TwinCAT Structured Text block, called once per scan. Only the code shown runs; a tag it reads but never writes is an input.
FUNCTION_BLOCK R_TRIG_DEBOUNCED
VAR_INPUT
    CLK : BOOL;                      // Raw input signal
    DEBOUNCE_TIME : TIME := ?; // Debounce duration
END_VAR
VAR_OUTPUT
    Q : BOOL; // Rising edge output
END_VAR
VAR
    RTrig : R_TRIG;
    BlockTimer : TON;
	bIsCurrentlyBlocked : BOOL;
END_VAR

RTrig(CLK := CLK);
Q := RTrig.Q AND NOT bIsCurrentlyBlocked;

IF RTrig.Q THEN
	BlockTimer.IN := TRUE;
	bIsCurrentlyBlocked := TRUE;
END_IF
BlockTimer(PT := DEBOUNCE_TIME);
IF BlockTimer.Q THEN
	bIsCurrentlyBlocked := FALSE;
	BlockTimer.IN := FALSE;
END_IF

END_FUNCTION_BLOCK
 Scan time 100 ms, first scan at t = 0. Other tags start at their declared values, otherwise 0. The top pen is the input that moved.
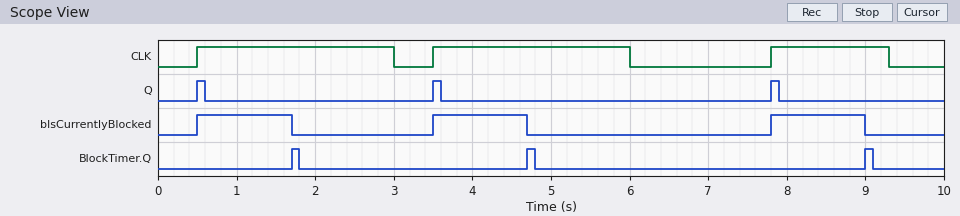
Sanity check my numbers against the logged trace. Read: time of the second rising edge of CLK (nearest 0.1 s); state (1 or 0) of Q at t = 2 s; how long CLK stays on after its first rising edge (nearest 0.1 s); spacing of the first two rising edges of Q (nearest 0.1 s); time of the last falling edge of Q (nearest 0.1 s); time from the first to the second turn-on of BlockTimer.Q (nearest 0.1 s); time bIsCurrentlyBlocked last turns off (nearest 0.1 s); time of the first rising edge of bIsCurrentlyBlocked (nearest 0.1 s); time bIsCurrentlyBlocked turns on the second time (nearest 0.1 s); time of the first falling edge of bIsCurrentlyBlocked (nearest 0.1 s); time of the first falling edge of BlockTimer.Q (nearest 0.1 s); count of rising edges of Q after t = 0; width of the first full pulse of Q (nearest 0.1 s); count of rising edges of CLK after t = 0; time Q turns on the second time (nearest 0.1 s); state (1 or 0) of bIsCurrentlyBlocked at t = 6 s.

3.5 s
0
2.5 s
3.0 s
7.9 s
3.0 s
9.0 s
0.5 s
3.5 s
1.7 s
1.8 s
3
0.1 s
3
3.5 s
0
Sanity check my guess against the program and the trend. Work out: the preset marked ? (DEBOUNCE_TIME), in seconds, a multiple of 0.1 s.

1.2 s
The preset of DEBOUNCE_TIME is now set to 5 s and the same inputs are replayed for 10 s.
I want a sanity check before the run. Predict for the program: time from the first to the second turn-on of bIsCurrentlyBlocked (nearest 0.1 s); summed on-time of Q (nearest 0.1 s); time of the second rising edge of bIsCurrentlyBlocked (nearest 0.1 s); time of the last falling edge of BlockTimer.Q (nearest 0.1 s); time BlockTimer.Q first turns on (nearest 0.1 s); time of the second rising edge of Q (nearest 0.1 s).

7.3 s
0.2 s
7.8 s
5.6 s
5.5 s
7.8 s
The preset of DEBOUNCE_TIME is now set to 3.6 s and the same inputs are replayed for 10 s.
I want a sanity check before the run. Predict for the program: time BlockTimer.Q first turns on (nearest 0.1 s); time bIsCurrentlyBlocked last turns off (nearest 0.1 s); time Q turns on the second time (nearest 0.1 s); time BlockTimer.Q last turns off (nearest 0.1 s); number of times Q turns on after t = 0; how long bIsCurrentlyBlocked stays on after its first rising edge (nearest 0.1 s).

4.1 s
4.1 s
7.8 s
4.2 s
2
3.6 s
